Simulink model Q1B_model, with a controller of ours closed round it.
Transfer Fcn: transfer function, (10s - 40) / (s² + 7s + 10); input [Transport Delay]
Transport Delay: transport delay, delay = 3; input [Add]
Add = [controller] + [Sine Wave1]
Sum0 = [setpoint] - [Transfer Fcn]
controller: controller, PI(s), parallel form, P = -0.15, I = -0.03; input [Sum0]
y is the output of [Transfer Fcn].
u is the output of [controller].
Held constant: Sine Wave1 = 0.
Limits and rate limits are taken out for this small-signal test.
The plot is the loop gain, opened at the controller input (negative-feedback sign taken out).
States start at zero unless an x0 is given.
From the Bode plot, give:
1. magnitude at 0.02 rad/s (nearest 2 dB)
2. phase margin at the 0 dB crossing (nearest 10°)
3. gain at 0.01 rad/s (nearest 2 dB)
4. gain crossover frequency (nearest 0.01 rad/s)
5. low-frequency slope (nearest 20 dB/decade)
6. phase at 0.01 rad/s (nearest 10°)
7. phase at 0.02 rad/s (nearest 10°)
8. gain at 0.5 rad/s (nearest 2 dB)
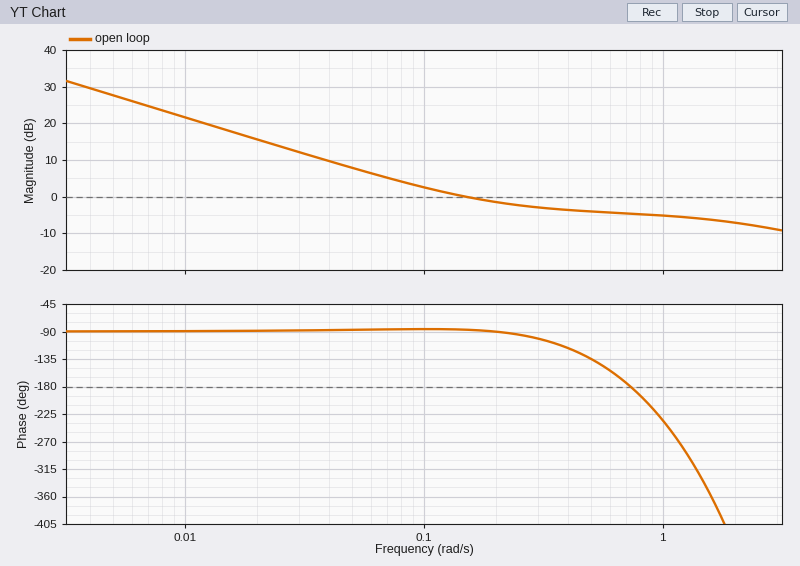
16 dB
90°
22 dB
0.15 rad/s
-20 dB/decade
-90°
-90°
-4 dB
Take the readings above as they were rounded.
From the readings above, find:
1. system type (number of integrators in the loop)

1
